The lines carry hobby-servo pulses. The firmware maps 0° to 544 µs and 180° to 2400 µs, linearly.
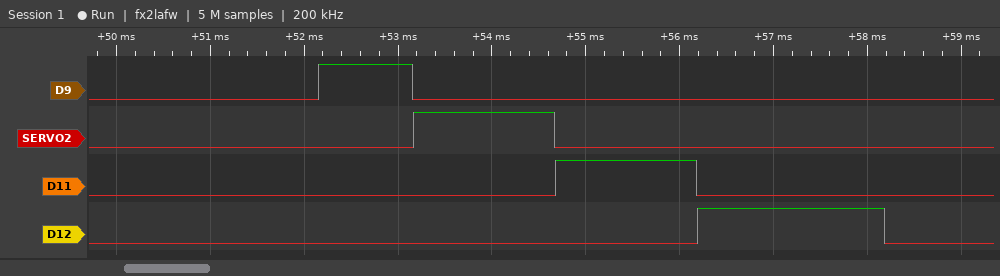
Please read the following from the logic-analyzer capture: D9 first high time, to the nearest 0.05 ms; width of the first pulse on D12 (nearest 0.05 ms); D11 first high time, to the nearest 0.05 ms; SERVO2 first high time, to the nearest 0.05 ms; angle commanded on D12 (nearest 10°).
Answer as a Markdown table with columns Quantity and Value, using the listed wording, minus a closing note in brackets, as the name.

| Quantity | Value |
|---|---|
| D9 first high time, to the nearest 0.05 ms | 1.00 ms |
| width of the first pulse on D12 | 2.00 ms |
| D11 first high time, to the nearest 0.05 ms | 1.50 ms |
| SERVO2 first high time, to the nearest 0.05 ms | 1.50 ms |
| angle commanded on D12 | 140° |
